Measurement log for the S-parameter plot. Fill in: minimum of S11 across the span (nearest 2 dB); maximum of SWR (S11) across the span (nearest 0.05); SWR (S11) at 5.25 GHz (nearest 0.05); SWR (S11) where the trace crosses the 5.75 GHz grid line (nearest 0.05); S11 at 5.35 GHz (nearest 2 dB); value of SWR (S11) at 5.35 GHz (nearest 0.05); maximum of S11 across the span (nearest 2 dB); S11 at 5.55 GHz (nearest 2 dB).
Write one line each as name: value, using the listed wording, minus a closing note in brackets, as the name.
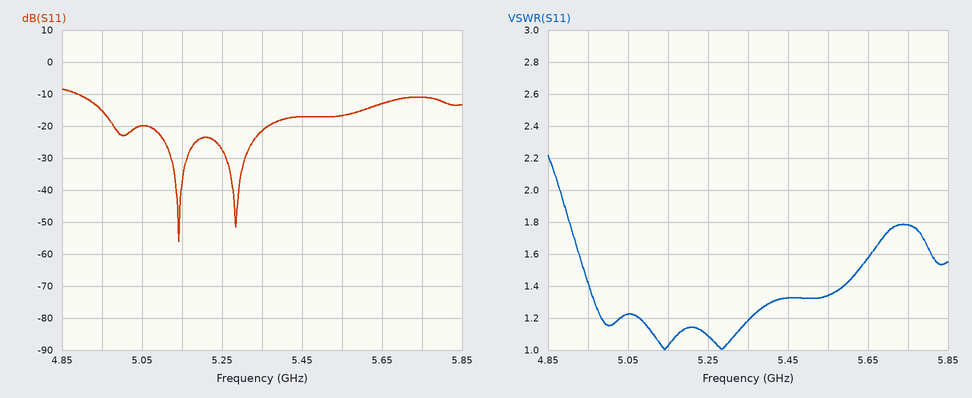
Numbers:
minimum of S11 across the span: -56 dB
maximum of SWR (S11) across the span: 2.20
SWR (S11) at 5.25 GHz: 1.10
SWR (S11) where the trace crosses the 5.75 GHz grid line: 1.80
S11 at 5.35 GHz: -22 dB
value of SWR (S11) at 5.35 GHz: 1.20
maximum of S11 across the span: -8 dB
S11 at 5.55 GHz: -16 dB
